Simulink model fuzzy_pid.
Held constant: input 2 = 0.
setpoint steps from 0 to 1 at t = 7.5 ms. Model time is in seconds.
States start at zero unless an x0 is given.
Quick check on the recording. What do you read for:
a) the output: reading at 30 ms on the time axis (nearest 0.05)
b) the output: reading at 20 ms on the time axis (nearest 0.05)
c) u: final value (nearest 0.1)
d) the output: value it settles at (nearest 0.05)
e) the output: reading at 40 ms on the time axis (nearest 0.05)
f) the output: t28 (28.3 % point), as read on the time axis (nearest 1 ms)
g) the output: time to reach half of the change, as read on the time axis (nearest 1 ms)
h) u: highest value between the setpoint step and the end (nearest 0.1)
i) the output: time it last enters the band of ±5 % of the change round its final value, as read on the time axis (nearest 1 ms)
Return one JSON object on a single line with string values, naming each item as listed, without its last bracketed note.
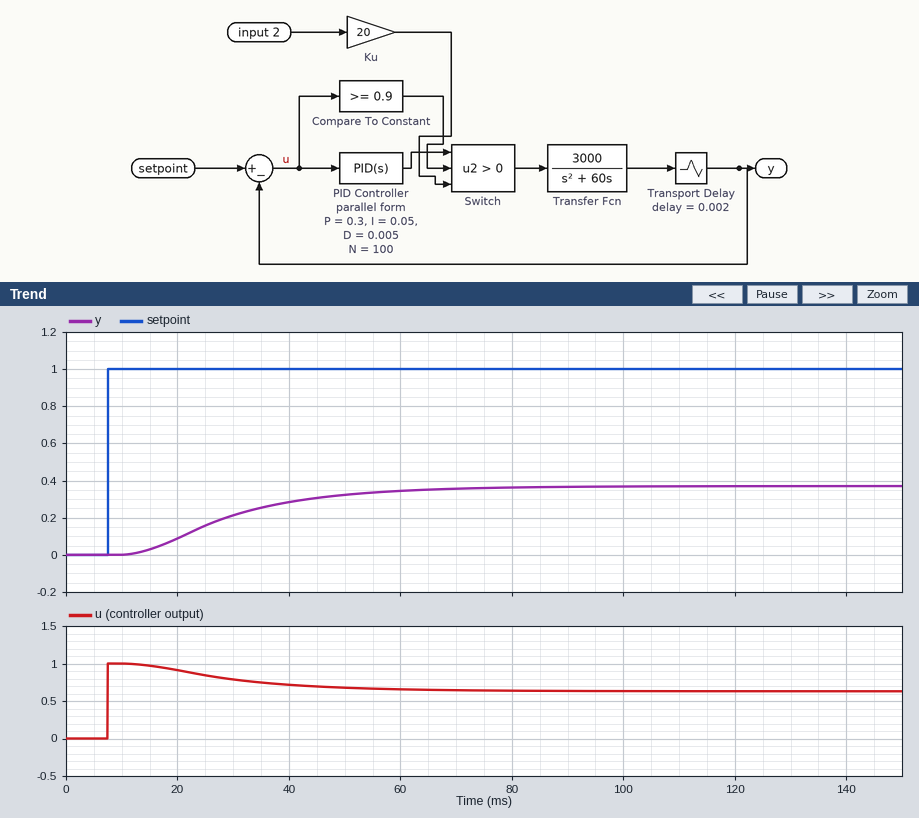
{"the output: reading at 30 ms on the time axis": "0.20", "the output: reading at 20 ms on the time axis": "0.10", "u: final value": "0.6", "the output: value it settles at": "0.35", "the output: reading at 40 ms on the time axis": "0.30", "the output: t28 (28.3 % point), as read on the time axis": "21 ms", "the output: time to reach half of the change, as read on the time axis": "27 ms", "u: highest value between the setpoint step and the end": "1.0", "the output: time it last enters the band of ±5 % of the change round its final value, as read on the time axis": "66 ms"}
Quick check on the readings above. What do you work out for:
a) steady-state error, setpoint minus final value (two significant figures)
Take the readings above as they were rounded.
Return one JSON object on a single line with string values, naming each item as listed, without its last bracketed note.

{"steady-state error, setpoint minus final value": "0.65"}
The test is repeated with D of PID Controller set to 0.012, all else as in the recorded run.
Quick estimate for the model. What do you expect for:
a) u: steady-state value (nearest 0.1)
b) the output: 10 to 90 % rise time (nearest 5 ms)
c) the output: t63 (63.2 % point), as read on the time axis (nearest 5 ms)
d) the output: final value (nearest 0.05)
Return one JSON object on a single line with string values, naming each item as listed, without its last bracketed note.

{"u: steady-state value": "0.5", "the output: 10 to 90 % rise time": "35 ms", "the output: t63 (63.2 % point), as read on the time axis": "30 ms", "the output: final value": "0.50"}
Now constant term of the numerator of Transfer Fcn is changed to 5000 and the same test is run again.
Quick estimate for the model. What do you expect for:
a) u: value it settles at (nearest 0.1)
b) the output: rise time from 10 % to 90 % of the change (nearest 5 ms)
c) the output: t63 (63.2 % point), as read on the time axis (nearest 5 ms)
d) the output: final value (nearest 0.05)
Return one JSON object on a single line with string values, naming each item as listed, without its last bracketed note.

{"u: value it settles at": "0.5", "the output: rise time from 10 % to 90 % of the change": "40 ms", "the output: t63 (63.2 % point), as read on the time axis": "30 ms", "the output: final value": "0.50"}
